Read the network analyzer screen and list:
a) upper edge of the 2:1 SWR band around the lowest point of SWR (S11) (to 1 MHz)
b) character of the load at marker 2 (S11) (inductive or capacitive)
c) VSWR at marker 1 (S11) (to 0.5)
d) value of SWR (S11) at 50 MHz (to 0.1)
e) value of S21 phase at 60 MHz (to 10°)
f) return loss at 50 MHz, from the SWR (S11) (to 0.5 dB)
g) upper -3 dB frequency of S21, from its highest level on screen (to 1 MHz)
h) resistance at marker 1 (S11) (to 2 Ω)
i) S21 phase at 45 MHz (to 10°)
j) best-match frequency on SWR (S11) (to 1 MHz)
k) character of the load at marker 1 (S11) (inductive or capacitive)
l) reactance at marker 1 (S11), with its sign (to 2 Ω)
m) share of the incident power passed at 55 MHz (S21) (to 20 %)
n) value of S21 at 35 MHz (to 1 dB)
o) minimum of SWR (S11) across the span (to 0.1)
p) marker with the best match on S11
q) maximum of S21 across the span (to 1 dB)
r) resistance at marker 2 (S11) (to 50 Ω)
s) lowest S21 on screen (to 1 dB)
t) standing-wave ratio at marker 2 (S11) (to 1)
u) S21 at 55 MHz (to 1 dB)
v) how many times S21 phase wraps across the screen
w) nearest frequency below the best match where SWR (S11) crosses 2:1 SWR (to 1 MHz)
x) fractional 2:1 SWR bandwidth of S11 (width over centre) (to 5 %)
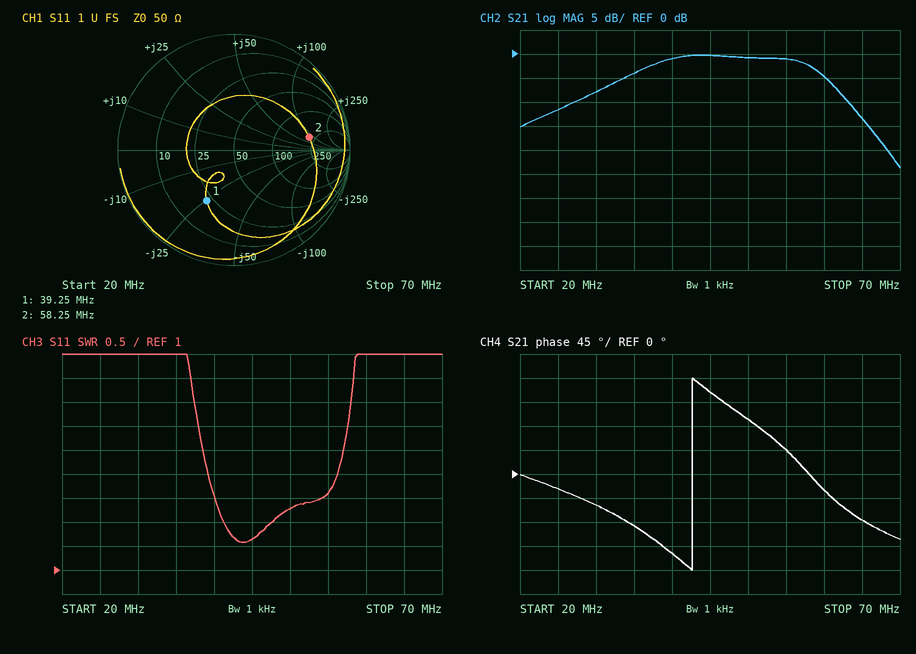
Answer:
48 MHz
inductive
3.0
2.3
-30°
8.0 dB
59 MHz
22 Ω
150°
44 MHz
capacitive
-26 Ω
80 %
-4 dB
1.6
marker 1
0 dB
200 Ω
-24 dB
5
-1 dB
1
41 MHz
15 %
